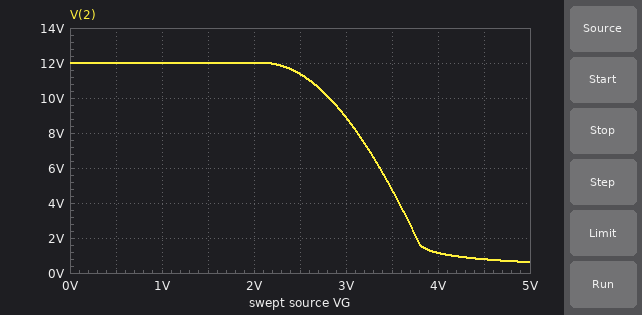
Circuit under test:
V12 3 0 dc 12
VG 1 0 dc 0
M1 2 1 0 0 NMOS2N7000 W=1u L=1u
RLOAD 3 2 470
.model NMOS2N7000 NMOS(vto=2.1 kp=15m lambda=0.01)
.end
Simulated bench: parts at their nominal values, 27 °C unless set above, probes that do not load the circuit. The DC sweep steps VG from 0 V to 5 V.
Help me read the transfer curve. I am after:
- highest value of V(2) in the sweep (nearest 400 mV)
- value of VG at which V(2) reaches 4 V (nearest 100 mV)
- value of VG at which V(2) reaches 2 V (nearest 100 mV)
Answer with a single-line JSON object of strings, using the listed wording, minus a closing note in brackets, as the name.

{"highest value of V(2) in the sweep": "12.0 V", "value of VG at which V(2) reaches 4 V": "3.6 V", "value of VG at which V(2) reaches 2 V": "3.8 V"}
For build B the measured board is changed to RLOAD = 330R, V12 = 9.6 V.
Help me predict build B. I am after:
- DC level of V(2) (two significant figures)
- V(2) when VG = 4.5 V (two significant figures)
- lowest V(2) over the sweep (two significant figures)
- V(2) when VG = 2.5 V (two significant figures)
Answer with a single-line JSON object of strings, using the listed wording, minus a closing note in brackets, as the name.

{"DC level of V(2)": "9.6 V", "V(2) when VG = 4.5 V": "890 mV", "lowest V(2) over the sweep": "700 mV", "V(2) when VG = 2.5 V": "9.2 V"}
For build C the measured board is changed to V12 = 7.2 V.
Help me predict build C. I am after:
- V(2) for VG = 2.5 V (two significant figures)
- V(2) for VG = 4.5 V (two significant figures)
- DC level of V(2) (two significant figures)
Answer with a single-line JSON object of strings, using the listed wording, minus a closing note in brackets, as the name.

{"V(2) for VG = 2.5 V": "6.6 V", "V(2) for VG = 4.5 V": "440 mV", "DC level of V(2)": "7.2 V"}
